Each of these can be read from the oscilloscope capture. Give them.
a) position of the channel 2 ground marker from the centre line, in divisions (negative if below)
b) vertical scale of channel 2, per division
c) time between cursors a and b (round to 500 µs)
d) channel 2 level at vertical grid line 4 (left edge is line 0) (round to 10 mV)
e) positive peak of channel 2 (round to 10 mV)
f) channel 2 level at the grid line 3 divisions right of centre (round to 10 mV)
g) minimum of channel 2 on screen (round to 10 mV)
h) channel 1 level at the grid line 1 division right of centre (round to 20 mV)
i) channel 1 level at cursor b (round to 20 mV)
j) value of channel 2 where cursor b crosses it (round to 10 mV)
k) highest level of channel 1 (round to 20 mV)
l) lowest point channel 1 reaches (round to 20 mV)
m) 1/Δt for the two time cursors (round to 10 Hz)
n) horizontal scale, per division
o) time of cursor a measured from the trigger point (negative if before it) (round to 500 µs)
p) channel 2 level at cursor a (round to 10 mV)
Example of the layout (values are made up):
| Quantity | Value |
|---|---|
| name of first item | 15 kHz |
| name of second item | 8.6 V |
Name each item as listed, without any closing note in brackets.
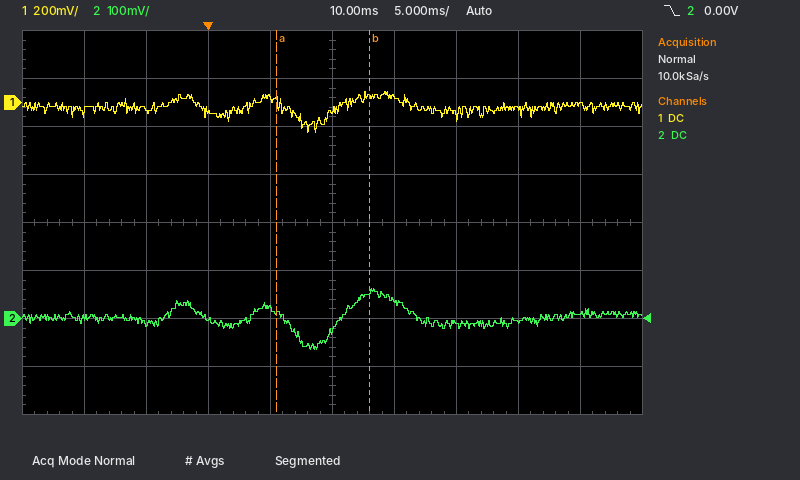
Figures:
| Quantity | Value |
|---|---|
| position of the channel 2 ground marker from the centre line, in divisions | -2.0 div |
| vertical scale of channel 2, per division | 100 mV |
| time between cursors a and b | 7.5 ms |
| channel 2 level at vertical grid line 4 (left edge is line 0) | 20 mV |
| positive peak of channel 2 | 60 mV |
| channel 2 level at the grid line 3 divisions right of centre | -10 mV |
| minimum of channel 2 on screen | -60 mV |
| channel 1 level at the grid line 1 division right of centre | 20 mV |
| channel 1 level at cursor b | 20 mV |
| value of channel 2 where cursor b crosses it | 60 mV |
| highest level of channel 1 | 40 mV |
| lowest point channel 1 reaches | -120 mV |
| 1/Δt for the two time cursors | 130 Hz |
| horizontal scale, per division | 5 ms |
| time of cursor a measured from the trigger point (negative if before it) | +5.5 ms |
| channel 2 level at cursor a | 10 mV |
